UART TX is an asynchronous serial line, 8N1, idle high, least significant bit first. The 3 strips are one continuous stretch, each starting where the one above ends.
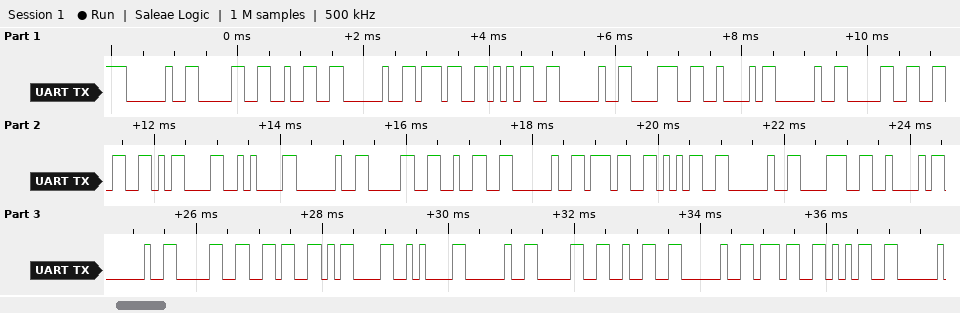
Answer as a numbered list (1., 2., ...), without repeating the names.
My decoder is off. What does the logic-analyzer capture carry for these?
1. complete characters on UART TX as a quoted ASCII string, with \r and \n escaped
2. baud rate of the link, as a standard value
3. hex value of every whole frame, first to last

1. " 02 75 8B 06\r\n 02 75 8B 06\r\n 02 75"
2. 9600 baud
3. 0x20 0x30 0x32 0x20 0x37 0x35 0x20 0x38 0x42 0x20 0x30 0x36 0x0D 0x0A 0x20 0x30 0x32 0x20 0x37 0x35 0x20 0x38 0x42 0x20 0x30 0x36 0x0D 0x0A 0x20 0x30 0x32 0x20 0x37 0x35
